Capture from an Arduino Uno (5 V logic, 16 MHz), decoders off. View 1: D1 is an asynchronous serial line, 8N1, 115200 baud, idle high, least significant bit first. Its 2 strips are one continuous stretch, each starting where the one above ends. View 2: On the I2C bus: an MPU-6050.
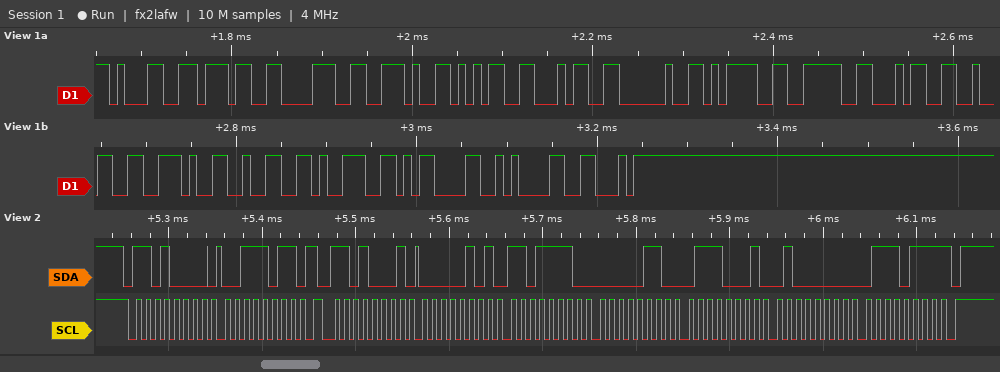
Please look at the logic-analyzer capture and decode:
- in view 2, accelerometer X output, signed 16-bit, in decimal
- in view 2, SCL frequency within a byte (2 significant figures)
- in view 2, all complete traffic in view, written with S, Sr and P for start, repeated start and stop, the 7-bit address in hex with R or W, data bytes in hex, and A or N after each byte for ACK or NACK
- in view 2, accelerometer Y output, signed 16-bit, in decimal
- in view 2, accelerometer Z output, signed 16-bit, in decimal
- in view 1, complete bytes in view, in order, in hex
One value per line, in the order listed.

1502
100 kHz
S 68W A 3B A Sr 68R A 05 A DE A 06 A 71 A 40 A 77 N P
1649
16503
0x31 0x37 0x38 0x2E 0x35 0x34 0x20 0x3D 0x3E 0x34 0x32 0x2E 0x32 0x39 0x0D 0x0A 0x46
